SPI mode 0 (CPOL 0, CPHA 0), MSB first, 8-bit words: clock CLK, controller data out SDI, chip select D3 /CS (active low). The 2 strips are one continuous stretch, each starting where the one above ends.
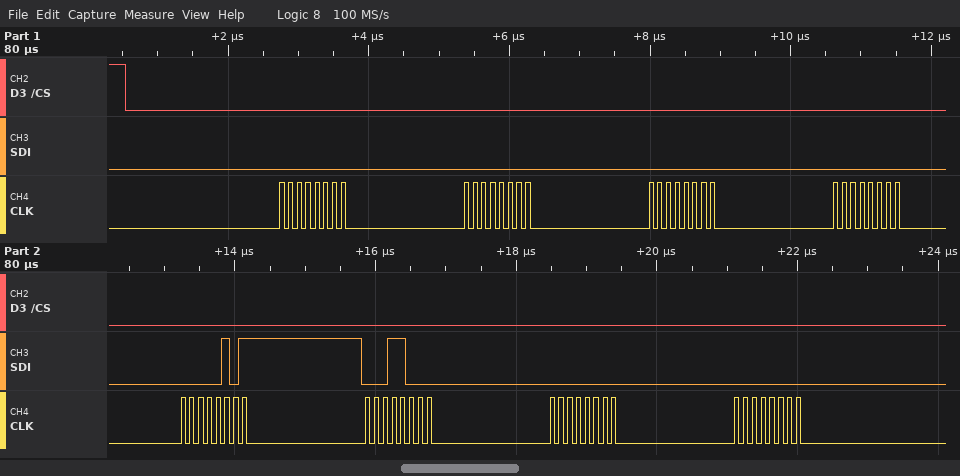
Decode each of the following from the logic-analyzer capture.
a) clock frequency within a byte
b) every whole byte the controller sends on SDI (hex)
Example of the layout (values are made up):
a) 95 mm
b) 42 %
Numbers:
a) 8 MHz
b) 00 00 00 00 05 18 00 00
